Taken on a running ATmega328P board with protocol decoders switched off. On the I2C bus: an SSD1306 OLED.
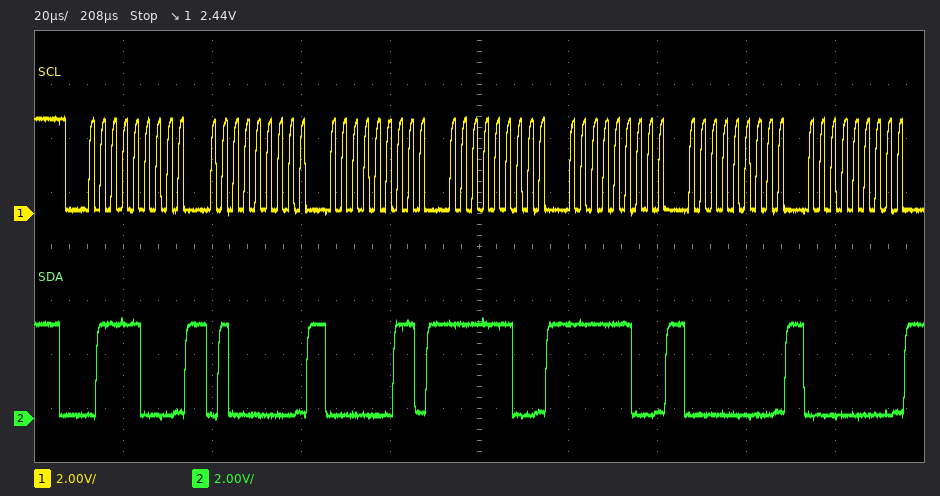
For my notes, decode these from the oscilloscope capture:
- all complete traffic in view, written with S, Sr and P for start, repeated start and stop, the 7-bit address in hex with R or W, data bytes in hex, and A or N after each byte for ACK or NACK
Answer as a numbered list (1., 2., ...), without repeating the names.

1. S 3CW A 40 A 03 A FC A FC A 00 A 00 A
